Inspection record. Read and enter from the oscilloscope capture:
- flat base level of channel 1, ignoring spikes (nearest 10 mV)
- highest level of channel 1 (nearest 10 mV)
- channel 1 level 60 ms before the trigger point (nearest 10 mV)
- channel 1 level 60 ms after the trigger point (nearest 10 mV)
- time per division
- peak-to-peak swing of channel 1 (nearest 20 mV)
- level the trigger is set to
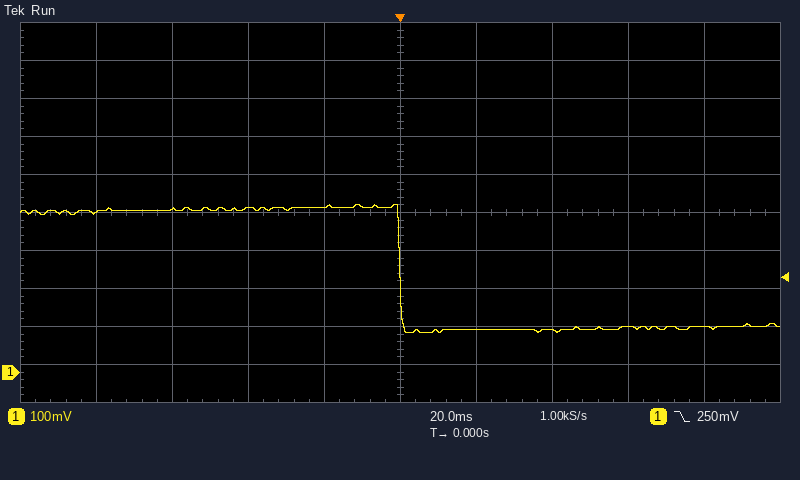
110 mV
440 mV
430 mV
120 mV
20 ms
340 mV
250 mV
